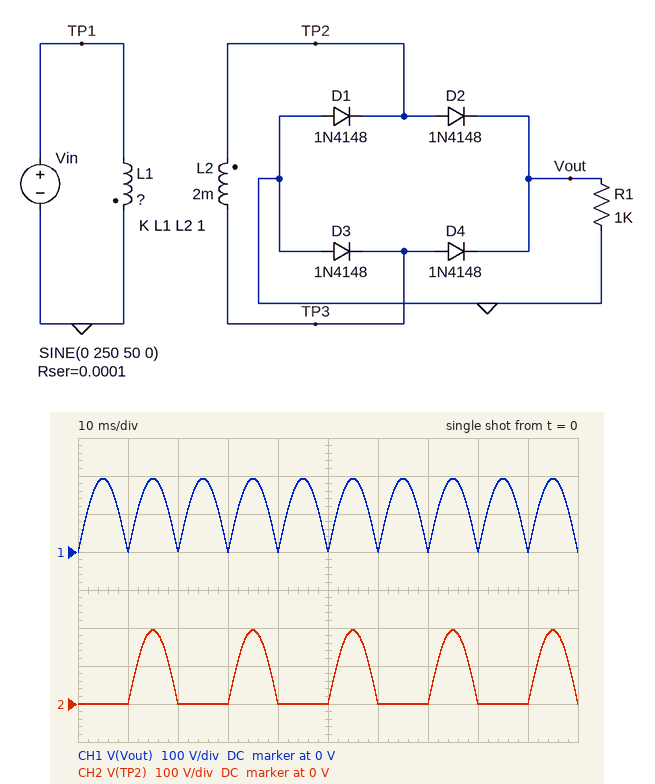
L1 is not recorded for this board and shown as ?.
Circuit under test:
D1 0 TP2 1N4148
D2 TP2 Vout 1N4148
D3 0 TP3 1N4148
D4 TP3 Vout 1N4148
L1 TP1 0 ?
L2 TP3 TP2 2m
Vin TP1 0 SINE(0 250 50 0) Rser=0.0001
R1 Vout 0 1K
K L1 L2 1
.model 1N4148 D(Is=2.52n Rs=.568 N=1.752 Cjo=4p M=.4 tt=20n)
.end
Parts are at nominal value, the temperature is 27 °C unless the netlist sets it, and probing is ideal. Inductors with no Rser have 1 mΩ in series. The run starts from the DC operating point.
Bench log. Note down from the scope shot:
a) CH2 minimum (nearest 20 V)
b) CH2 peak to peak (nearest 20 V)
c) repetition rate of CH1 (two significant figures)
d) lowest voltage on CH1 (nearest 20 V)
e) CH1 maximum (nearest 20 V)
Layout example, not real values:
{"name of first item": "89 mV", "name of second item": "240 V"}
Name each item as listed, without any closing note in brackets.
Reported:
{"CH2 minimum": "0 V", "CH2 peak to peak": "200 V", "repetition rate of CH1": "100 Hz", "lowest voltage on CH1": "0 V", "CH1 maximum": "200 V"}
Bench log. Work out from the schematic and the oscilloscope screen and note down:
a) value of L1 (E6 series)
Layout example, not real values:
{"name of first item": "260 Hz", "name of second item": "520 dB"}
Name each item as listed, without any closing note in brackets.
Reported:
{"value of L1": "3.3 mH"}
